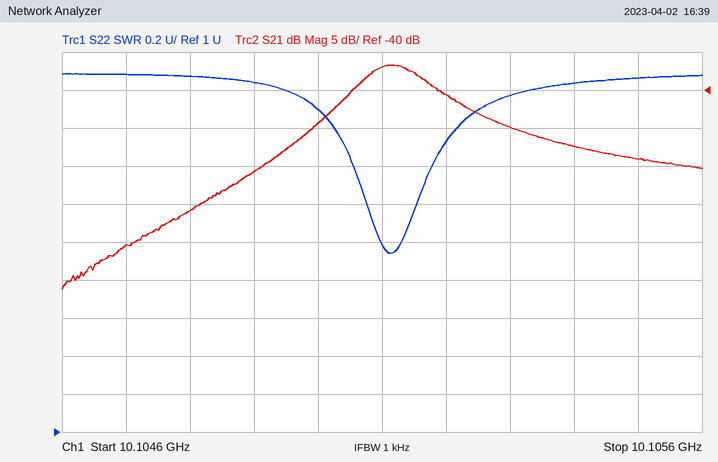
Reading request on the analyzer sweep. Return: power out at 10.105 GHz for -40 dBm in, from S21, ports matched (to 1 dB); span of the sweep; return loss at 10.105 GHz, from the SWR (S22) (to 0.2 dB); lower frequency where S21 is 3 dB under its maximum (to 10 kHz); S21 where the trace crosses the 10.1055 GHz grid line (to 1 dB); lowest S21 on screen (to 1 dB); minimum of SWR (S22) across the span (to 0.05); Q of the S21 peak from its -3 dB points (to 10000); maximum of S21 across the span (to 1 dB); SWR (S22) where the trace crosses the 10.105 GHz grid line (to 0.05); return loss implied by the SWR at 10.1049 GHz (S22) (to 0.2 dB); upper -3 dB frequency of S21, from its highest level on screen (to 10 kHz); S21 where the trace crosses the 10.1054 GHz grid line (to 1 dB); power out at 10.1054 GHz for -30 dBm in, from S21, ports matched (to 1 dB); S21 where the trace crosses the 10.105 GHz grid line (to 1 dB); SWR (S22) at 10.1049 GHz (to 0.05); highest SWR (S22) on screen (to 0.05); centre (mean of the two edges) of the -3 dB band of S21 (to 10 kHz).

-84 dBm
1 MHz
6.8 dB
10.10506 GHz
-49 dB
-66 dB
1.95
80000
-37 dB
2.70
6.4 dB
10.10518 GHz
-47 dB
-77 dBm
-44 dB
2.85
2.90
10.10512 GHz
